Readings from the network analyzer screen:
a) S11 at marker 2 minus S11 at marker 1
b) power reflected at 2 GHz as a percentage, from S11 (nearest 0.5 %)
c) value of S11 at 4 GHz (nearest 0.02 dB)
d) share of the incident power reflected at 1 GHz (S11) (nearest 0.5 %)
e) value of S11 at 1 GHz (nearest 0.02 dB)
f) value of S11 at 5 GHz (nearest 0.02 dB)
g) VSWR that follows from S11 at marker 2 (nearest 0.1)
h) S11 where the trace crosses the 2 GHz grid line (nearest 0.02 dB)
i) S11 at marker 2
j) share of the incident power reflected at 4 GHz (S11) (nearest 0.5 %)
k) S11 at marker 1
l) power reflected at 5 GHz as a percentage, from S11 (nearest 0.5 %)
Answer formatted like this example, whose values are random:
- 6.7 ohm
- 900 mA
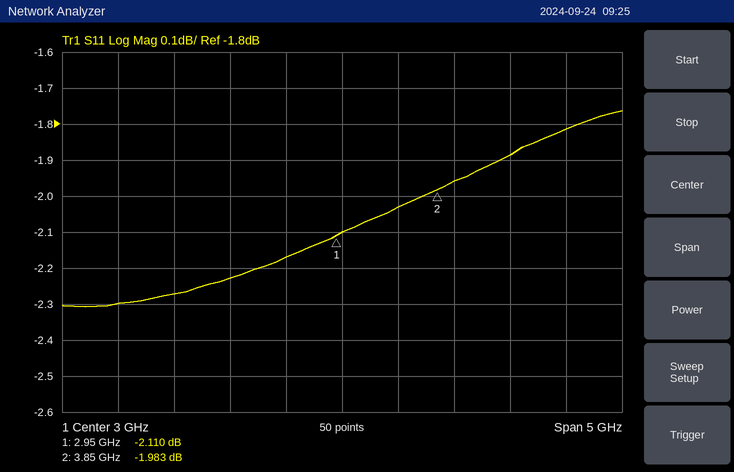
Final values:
- 0.127 dB
- 60.0 %
- -1.96 dB
- 59.0 %
- -2.30 dB
- -1.82 dB
- 8.8
- -2.22 dB
- -1.983 dB
- 63.5 %
- -2.110 dB
- 66.0 %
